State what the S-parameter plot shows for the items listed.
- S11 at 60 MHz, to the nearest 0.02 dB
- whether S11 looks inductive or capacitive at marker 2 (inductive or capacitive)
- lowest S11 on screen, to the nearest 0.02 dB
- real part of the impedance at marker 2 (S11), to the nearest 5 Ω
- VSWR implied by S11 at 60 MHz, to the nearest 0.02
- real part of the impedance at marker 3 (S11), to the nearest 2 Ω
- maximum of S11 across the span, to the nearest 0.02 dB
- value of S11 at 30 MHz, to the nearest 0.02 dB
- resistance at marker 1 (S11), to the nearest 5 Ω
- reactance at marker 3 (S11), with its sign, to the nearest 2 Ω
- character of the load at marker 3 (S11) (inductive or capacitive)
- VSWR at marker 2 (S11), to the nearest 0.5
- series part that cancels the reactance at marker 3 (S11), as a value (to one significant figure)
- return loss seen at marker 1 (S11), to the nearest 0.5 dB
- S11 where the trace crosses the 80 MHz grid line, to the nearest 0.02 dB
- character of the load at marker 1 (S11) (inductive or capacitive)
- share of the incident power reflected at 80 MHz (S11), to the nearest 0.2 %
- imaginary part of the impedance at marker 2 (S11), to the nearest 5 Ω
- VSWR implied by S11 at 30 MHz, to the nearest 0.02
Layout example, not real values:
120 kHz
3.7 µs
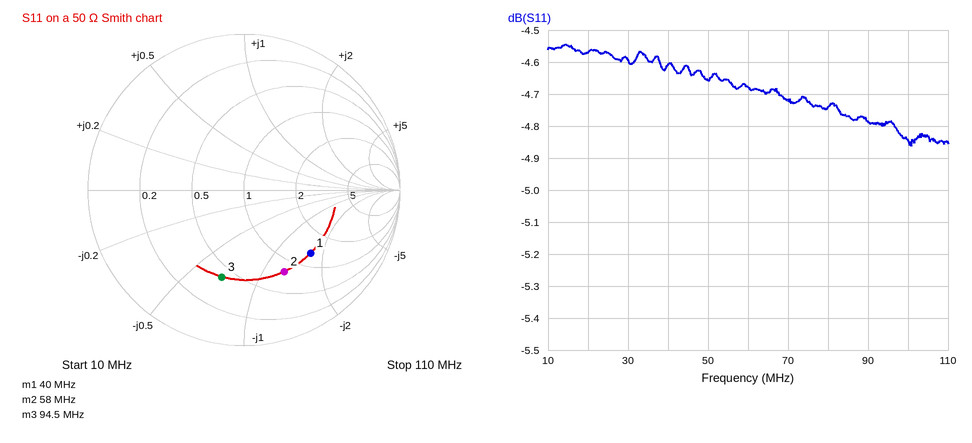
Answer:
-4.68 dB
capacitive
-4.86 dB
40 Ω
3.80
20 Ω
-4.54 dB
-4.60 dB
65 Ω
-34 Ω
capacitive
4.0
60 nH
4.5 dB
-4.74 dB
capacitive
33.6 %
-65 Ω
3.86
